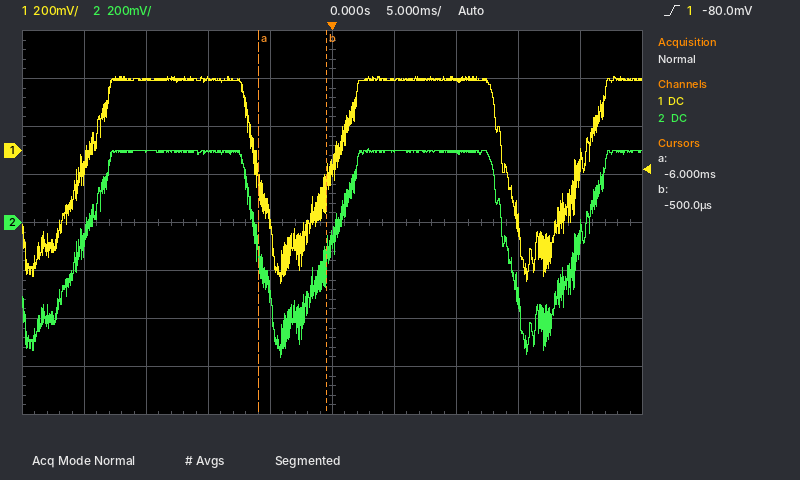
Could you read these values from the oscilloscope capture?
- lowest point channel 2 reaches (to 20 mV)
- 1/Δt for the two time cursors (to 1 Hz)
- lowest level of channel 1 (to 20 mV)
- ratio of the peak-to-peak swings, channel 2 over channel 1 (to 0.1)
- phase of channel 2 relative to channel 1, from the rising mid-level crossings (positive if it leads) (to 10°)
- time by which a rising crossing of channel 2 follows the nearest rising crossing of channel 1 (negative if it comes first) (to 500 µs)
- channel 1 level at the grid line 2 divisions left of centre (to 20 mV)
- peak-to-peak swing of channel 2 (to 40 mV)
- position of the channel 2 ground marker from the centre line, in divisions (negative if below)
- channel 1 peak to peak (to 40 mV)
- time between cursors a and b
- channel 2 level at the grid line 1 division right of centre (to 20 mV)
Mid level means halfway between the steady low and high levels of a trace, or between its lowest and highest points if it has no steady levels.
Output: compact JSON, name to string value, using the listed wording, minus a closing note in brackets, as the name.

{"lowest point channel 2 reaches": "-560 mV", "1/Δt for the two time cursors": "182 Hz", "lowest level of channel 1": "-560 mV", "ratio of the peak-to-peak swings, channel 2 over channel 1": "1.0", "phase of channel 2 relative to channel 1, from the rising mid-level crossings (positive if it leads)": "0°", "time by which a rising crossing of channel 2 follows the nearest rising crossing of channel 1 (negative if it comes first)": "0.0 ms", "channel 1 level at the grid line 2 divisions left of centre": "300 mV", "peak-to-peak swing of channel 2": "880 mV", "position of the channel 2 ground marker from the centre line, in divisions": "0.0 div", "channel 1 peak to peak": "880 mV", "time between cursors a and b": "5.5 ms", "channel 2 level at the grid line 1 division right of centre": "300 mV"}
